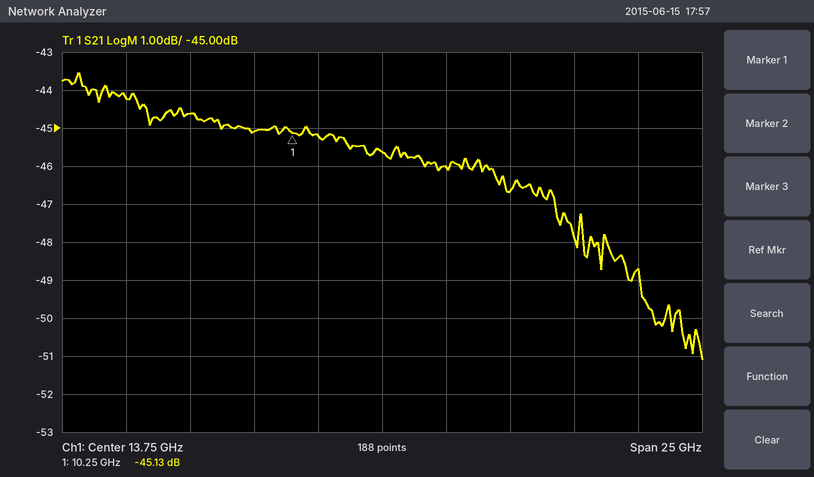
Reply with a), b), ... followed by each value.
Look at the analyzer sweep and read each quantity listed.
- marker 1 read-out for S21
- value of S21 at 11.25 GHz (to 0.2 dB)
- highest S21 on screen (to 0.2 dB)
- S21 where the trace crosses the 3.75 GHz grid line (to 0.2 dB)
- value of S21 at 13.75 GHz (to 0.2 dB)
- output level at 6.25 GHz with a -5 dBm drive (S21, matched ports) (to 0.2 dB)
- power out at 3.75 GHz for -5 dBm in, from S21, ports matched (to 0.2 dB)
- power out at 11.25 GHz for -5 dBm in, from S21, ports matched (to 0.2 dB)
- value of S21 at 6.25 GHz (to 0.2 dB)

a) -45.13 dB
b) -45.2 dB
c) -43.6 dB
d) -44.2 dB
e) -45.6 dB
f) -49.6 dBm
g) -49.2 dBm
h) -50.2 dBm
i) -44.6 dB
